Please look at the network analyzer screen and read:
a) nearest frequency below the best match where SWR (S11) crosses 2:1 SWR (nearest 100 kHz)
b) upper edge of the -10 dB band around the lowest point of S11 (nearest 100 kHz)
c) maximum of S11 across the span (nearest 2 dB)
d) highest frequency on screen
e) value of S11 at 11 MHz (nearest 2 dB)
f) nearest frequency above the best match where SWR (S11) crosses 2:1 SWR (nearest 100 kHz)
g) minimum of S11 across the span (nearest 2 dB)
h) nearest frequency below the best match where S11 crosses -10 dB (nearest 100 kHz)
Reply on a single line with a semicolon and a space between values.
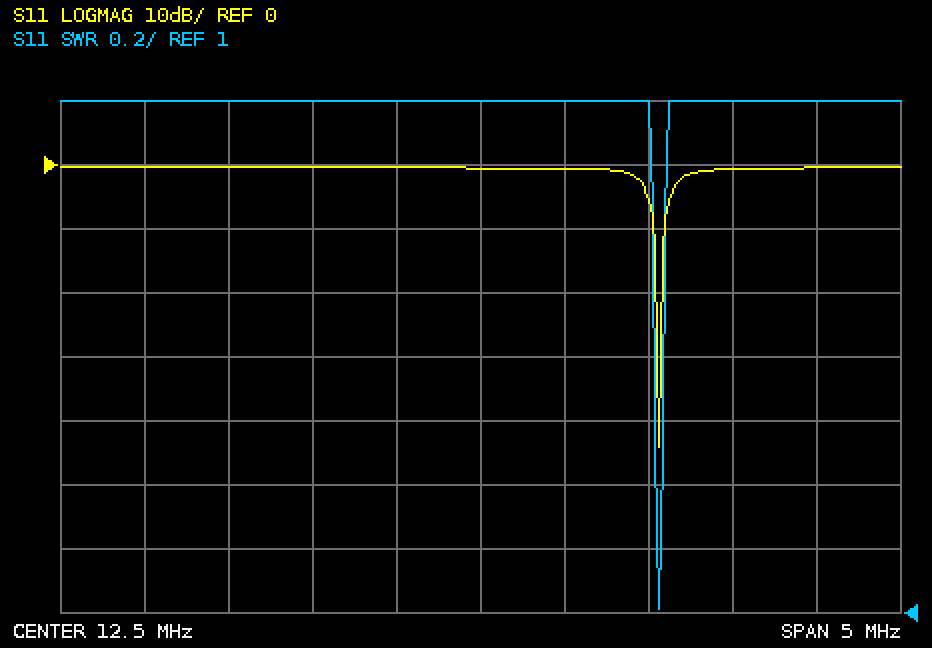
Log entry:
13.5 MHz; 13.6 MHz; 0 dB; 15 MHz; 0 dB; 13.6 MHz; -44 dB; 13.5 MHz
